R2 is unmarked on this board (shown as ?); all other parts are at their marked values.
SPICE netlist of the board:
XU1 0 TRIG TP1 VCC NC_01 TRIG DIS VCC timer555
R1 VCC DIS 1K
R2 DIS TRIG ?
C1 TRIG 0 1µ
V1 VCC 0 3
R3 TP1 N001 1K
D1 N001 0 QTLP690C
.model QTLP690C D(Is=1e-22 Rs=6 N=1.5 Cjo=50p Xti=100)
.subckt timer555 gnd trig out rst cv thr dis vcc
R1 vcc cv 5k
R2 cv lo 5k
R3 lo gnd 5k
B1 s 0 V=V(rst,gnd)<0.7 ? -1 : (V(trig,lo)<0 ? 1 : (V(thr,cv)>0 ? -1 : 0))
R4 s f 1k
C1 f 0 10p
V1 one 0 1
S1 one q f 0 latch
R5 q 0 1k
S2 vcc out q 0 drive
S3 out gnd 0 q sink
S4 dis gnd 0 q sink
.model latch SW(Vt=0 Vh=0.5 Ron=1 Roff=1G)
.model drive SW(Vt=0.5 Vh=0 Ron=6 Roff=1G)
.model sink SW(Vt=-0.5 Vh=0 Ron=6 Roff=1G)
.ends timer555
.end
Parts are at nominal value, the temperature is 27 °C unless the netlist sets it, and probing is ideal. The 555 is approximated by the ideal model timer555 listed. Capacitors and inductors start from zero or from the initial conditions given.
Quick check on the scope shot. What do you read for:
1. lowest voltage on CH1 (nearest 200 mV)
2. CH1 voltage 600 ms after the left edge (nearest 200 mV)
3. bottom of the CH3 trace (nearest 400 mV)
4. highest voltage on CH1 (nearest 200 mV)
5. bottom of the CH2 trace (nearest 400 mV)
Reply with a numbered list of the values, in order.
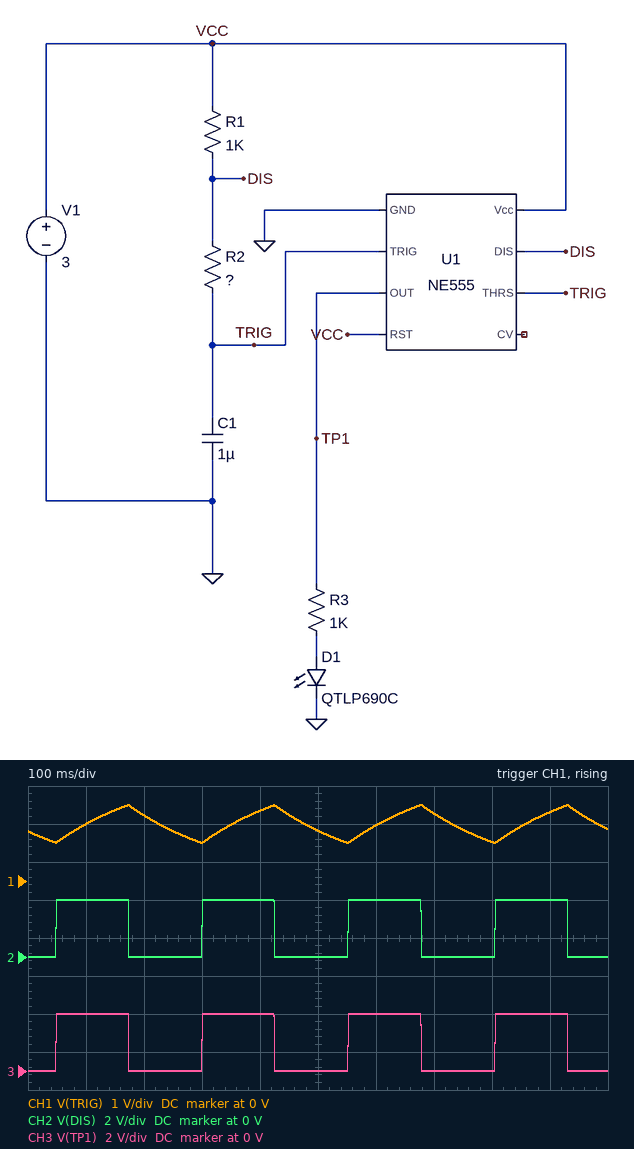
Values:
1. 1.0 V
2. 1.4 V
3. 0 V
4. 2.0 V
5. 0 V
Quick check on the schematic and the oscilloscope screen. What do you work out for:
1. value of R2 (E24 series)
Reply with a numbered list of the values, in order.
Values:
1. 180 kΩ
